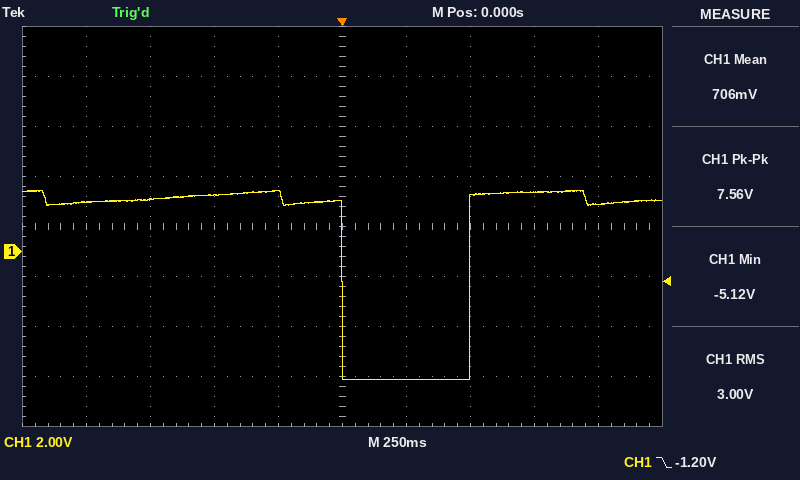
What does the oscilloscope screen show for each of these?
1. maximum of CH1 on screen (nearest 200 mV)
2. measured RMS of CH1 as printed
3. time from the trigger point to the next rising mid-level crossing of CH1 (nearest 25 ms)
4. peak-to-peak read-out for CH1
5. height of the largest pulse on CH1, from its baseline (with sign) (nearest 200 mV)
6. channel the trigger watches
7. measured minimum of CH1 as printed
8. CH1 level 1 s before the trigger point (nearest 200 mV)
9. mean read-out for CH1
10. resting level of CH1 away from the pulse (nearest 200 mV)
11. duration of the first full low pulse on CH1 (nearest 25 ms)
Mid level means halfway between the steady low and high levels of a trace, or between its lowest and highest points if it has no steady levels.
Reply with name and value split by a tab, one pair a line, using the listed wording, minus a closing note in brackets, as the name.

maximum of CH1 on screen	2.4 V
measured RMS of CH1 as printed	3.00 V
time from the trigger point to the next rising mid-level crossing of CH1	500 ms
peak-to-peak read-out for CH1	7.56 V
height of the largest pulse on CH1, from its baseline (with sign)	-7.2 V
channel the trigger watches	CH1
measured minimum of CH1 as printed	-5.12 V
CH1 level 1 s before the trigger point	2.0 V
mean read-out for CH1	706 mV
resting level of CH1 away from the pulse	2.0 V
duration of the first full low pulse on CH1	500 ms
